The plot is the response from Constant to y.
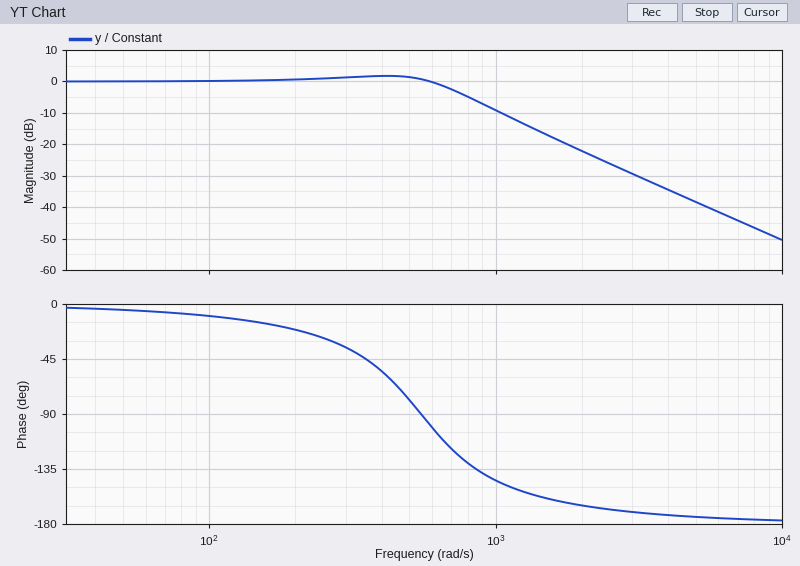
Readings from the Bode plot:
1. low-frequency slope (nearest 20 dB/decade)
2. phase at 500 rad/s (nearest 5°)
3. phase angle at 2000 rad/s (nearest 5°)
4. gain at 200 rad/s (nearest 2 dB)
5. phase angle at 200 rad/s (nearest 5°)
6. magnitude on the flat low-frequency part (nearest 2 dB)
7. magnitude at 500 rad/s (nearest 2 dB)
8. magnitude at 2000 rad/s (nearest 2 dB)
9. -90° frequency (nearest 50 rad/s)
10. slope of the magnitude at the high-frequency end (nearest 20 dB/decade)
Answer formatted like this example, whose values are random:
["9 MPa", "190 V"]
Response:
["0 dB/decade", "-80°", "-165°", "0 dB", "-20°", "0 dB", "2 dB", "-22 dB", "550 rad/s", "-40 dB/decade"]
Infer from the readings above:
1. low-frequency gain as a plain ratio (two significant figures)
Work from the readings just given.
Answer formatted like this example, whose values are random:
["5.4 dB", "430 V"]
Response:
["1.0"]
